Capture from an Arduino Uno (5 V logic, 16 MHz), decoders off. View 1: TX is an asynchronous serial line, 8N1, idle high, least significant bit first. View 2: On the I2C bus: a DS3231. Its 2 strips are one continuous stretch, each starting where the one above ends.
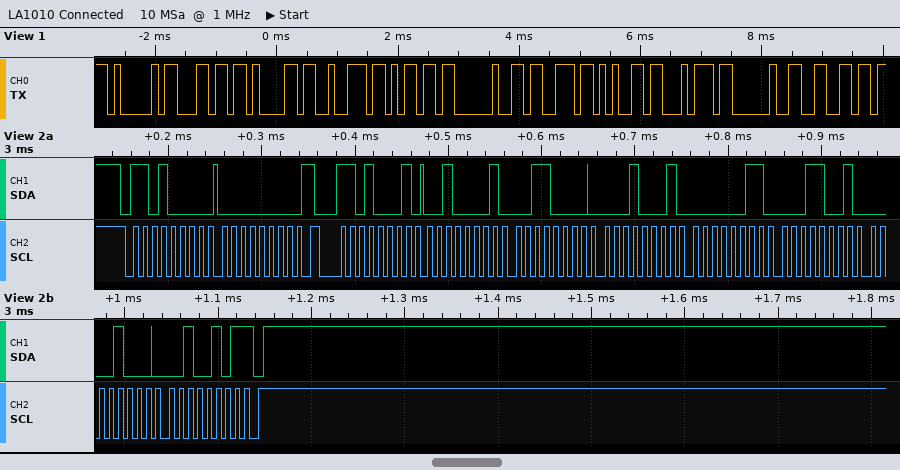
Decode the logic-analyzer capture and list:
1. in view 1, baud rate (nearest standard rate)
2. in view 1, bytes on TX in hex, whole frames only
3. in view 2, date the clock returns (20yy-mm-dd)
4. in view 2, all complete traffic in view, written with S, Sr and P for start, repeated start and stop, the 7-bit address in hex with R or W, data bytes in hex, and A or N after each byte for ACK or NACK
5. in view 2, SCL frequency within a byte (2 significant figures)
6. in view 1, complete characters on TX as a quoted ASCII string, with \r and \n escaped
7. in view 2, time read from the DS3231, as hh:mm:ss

9600 baud
41 6C 61 72 6D 20 73 65 74 20 66
2025-08-19
S 68W A 00 A Sr 68R A 21 A 30 A 11 A 03 A 19 A 08 A 25 N P
100 kHz
"Alarm set f"
11:30:21
